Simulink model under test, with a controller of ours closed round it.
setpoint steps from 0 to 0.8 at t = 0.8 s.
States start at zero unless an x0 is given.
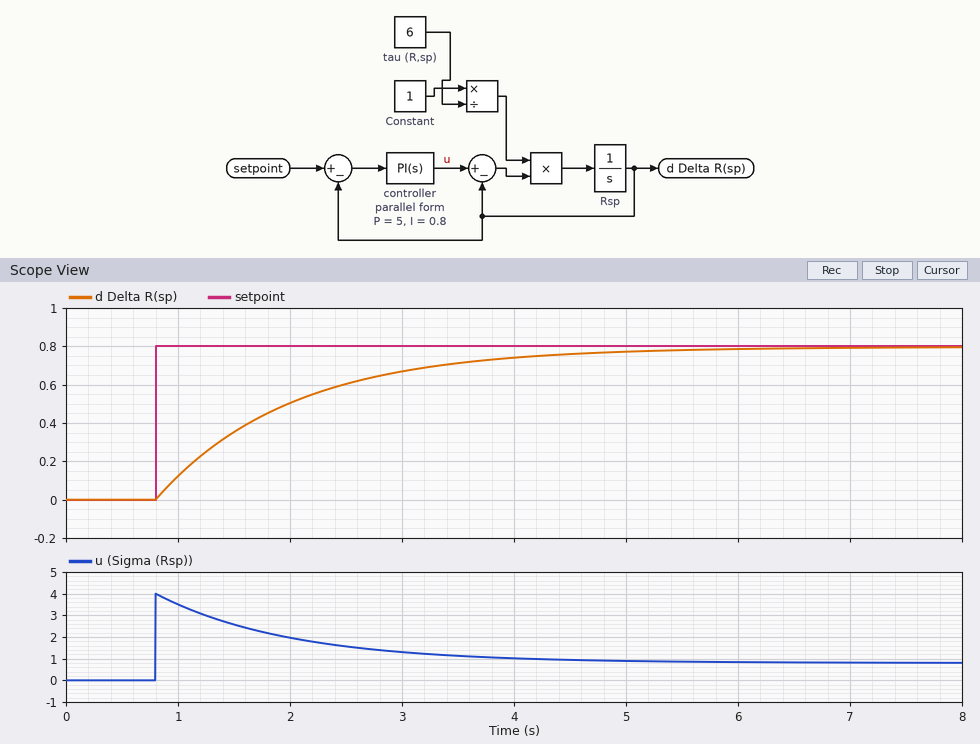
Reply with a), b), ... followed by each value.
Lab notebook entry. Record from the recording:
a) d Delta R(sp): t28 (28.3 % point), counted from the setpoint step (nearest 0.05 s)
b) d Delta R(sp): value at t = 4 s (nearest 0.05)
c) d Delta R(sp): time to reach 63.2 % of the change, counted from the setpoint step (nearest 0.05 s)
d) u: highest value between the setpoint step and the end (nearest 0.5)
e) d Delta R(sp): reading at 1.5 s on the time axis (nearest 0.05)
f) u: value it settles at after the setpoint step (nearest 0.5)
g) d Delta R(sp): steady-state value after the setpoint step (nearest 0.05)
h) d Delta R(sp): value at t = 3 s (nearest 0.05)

a) 0.40 s
b) 0.75
c) 1.20 s
d) 4.0
e) 0.35
f) 1.0
g) 0.80
h) 0.65
